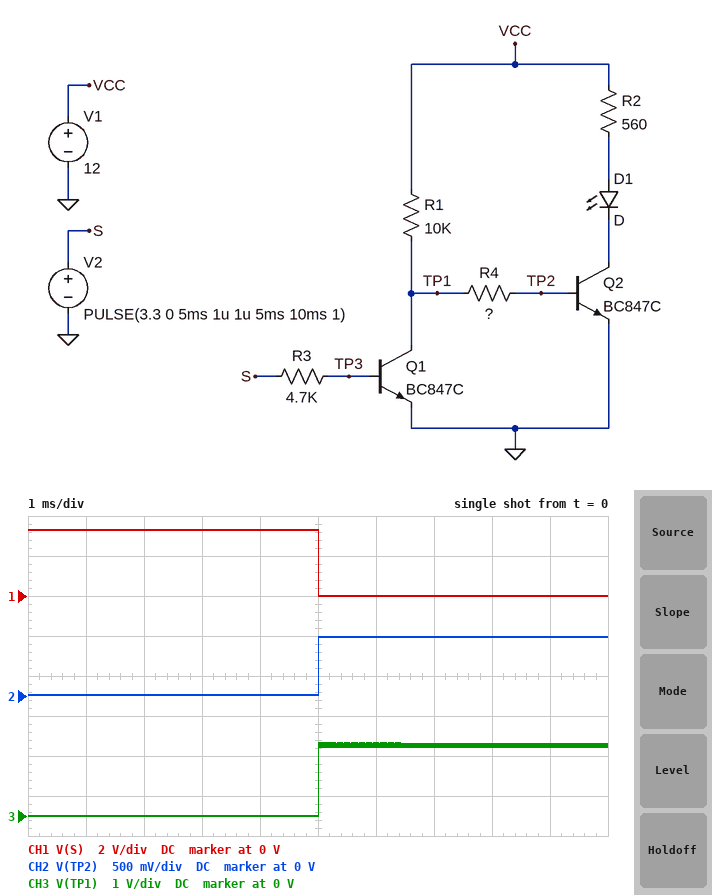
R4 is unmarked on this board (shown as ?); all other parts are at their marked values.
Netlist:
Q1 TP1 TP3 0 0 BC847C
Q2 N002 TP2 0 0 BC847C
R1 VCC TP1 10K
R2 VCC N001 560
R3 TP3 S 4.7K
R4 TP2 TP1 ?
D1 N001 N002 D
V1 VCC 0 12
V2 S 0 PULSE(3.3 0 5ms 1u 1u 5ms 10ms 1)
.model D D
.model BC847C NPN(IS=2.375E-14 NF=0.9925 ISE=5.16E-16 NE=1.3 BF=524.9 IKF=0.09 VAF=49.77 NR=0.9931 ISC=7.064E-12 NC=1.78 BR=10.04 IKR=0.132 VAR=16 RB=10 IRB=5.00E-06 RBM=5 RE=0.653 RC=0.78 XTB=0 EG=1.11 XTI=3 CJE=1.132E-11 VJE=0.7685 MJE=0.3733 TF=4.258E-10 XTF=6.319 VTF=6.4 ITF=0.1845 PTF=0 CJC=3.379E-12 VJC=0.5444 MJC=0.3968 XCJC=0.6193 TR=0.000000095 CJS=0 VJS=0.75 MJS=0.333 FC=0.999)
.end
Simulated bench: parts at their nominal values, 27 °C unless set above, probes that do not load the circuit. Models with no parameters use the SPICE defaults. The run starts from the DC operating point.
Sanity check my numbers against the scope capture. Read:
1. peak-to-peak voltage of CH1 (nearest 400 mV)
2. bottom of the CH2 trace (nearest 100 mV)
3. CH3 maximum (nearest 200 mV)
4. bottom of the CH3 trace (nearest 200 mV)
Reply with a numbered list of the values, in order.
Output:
1. 3.2 V
2. 0 V
3. 1.8 V
4. 0 V
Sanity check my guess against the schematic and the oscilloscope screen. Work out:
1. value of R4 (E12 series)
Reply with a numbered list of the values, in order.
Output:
1. 1 kΩ
